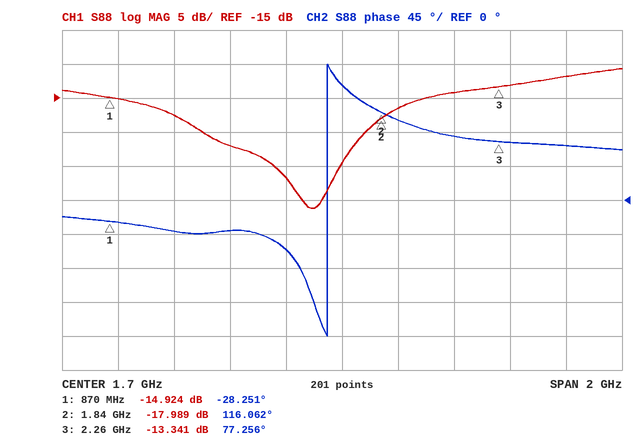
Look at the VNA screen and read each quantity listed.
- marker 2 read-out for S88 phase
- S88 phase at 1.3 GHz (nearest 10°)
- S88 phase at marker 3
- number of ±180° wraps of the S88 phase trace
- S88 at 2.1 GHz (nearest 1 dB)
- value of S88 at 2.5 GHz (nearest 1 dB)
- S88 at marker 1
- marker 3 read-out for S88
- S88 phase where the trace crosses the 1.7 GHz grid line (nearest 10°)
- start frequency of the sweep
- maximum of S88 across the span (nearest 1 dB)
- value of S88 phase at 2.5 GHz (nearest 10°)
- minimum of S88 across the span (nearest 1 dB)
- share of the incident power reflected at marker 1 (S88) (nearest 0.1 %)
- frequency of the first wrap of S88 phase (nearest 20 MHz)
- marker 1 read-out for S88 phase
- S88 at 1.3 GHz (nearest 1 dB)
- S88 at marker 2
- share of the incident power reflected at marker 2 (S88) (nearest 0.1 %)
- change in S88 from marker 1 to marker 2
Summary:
116.062°
-40°
77.256°
1
-14 dB
-12 dB
-14.924 dB
-13.341 dB
150°
700 MHz
-11 dB
70°
-31 dB
3.2 %
1.64 GHz
-28.251°
-22 dB
-17.989 dB
1.6 %
-3.065 dB
